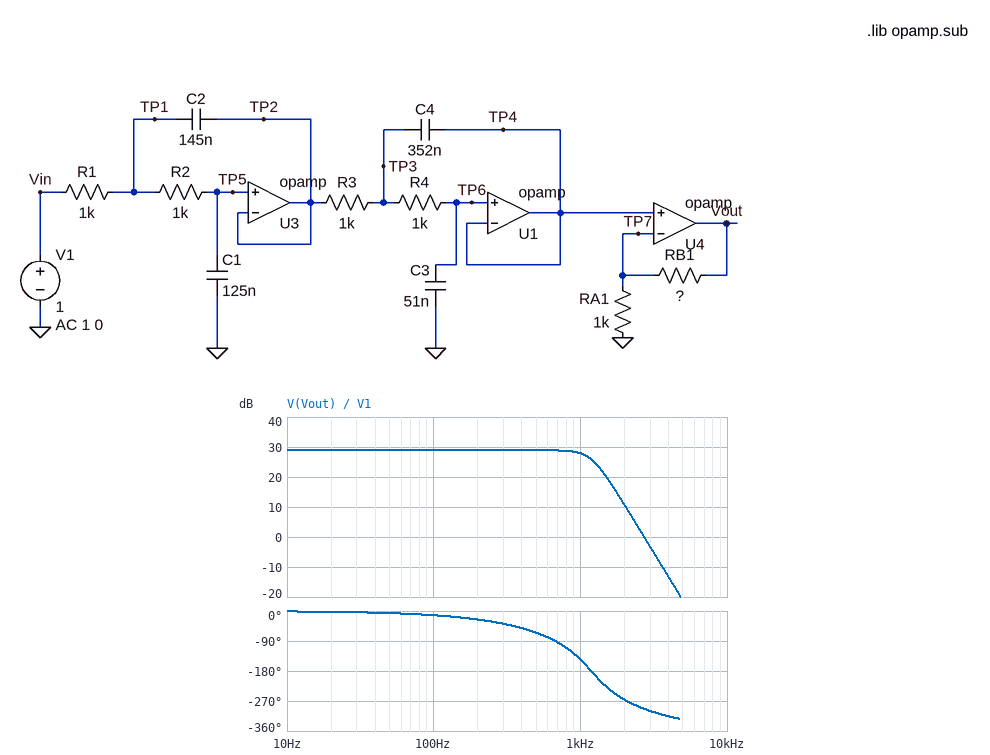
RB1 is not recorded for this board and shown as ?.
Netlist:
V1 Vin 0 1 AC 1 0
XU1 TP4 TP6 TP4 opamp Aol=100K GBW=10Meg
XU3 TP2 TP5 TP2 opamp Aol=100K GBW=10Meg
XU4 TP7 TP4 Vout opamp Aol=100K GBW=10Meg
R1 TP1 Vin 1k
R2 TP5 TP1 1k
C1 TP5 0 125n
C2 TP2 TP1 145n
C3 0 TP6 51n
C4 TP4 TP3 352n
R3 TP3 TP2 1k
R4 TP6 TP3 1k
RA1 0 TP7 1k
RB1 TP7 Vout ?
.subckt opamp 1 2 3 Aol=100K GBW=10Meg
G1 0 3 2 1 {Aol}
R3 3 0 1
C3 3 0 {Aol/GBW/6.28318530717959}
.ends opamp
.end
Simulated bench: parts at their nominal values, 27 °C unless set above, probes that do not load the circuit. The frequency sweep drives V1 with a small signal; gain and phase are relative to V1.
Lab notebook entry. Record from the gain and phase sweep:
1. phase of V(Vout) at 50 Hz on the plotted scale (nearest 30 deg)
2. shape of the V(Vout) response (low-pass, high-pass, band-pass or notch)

0 deg
low-pass
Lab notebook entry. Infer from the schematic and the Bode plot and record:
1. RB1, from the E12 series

27 kΩ
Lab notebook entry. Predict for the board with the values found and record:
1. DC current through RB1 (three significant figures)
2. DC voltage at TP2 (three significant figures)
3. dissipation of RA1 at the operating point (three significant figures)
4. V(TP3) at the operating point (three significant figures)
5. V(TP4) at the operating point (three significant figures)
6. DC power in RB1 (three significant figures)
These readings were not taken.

1.00 mA
1.00 V
999 µW
1.00 V
1.00 V
27.0 mW
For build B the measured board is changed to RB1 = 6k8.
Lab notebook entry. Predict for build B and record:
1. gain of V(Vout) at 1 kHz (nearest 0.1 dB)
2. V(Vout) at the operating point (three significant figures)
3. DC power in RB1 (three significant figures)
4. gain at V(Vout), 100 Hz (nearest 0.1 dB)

16.8 dB
7.80 V
6.80 mW
17.8 dB
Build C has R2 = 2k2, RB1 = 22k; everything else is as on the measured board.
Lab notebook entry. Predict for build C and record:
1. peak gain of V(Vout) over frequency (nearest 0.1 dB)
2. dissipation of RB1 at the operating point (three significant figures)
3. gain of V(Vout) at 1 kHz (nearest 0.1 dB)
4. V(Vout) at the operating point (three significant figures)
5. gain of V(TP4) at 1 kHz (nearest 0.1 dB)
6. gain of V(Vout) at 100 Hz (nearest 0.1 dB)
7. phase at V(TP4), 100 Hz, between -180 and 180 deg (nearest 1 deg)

27.2 dB
22.0 mW
22.1 dB
23.0 V
-5.2 dB
27.1 dB
-18 deg
